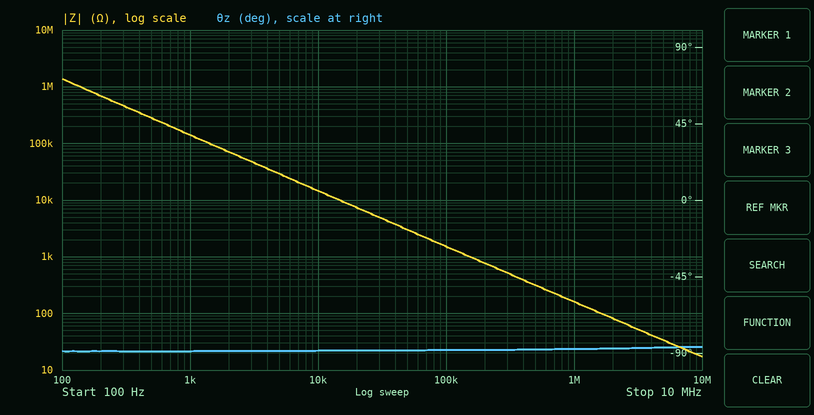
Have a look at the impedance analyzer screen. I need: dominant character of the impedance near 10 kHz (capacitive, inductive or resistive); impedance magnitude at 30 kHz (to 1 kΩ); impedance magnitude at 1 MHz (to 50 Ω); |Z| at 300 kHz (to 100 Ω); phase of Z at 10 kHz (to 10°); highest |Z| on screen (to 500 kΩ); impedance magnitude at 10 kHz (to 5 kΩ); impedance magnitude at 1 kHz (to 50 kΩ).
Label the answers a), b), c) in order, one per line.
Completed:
a) capacitive
b) 5 kΩ
c) 150 Ω
d) 500 Ω
e) -90°
f) 1.5 MΩ
g) 15 kΩ
h) 150 kΩ
